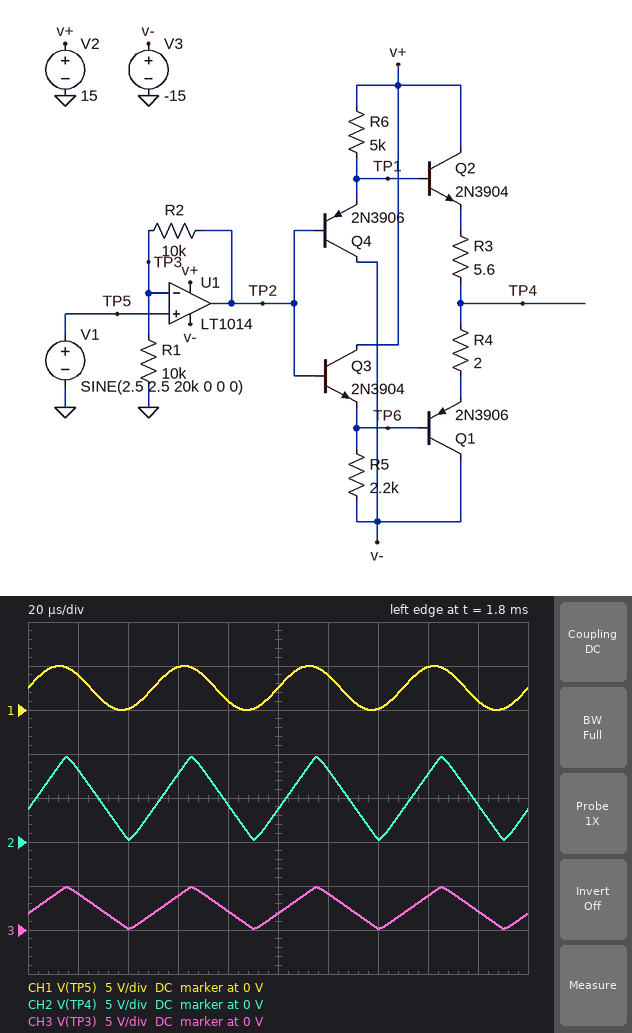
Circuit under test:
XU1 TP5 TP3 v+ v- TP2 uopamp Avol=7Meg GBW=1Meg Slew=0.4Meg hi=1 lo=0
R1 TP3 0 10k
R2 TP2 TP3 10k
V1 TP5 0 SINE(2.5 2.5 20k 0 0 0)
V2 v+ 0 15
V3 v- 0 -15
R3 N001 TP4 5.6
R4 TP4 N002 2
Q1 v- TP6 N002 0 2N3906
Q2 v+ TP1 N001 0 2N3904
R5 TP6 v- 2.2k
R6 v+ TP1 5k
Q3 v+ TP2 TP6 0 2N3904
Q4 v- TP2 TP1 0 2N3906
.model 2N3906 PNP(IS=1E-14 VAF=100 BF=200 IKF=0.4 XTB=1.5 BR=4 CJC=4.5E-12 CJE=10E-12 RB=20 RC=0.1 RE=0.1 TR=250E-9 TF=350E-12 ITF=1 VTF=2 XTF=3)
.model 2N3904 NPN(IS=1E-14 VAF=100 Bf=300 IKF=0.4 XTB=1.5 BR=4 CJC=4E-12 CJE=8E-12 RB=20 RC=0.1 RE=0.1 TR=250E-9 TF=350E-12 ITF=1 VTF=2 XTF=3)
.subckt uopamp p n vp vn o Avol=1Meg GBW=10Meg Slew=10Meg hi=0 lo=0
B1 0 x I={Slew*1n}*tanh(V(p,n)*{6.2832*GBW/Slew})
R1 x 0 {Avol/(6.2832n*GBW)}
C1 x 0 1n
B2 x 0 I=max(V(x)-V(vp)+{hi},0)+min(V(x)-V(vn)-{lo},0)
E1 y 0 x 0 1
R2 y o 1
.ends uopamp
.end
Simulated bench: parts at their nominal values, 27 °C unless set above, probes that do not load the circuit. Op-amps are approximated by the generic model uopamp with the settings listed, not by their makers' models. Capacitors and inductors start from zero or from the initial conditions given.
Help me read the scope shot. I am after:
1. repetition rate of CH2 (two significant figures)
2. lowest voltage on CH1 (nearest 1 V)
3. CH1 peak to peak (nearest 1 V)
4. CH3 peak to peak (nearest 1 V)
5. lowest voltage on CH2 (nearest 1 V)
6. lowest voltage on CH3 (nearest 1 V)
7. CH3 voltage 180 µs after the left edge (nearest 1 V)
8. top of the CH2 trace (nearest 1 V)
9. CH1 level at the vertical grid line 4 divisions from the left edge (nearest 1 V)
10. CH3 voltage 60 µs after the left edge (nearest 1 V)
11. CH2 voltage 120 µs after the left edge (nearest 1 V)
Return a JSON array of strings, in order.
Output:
["20 kHz", "0 V", "5 V", "5 V", "0 V", "0 V", "2 V", "10 V", "1 V", "4 V", "8 V"]
